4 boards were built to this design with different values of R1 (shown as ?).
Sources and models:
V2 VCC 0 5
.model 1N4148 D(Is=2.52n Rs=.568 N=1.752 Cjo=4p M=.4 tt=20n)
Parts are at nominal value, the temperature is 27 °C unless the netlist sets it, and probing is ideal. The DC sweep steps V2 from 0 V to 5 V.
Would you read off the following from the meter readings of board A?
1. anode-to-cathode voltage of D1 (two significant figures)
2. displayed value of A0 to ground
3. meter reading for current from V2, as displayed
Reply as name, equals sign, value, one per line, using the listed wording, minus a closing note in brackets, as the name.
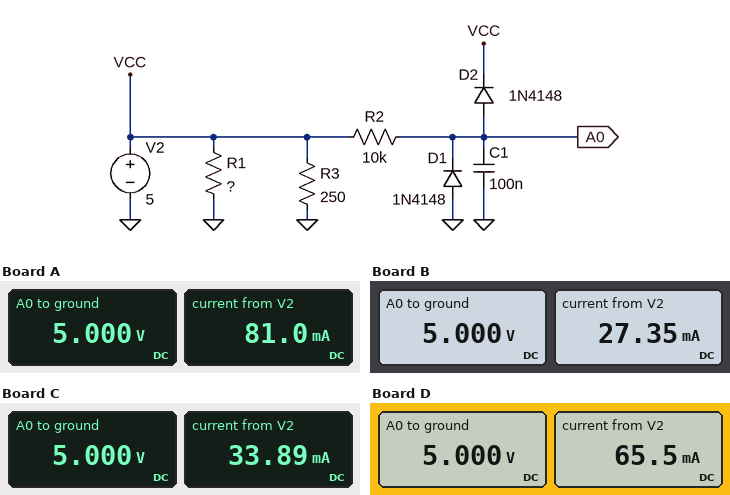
anode-to-cathode voltage of D1 = -5.0 V
displayed value of A0 to ground = 5.000 V
meter reading for current from V2, as displayed = 81.0 mA
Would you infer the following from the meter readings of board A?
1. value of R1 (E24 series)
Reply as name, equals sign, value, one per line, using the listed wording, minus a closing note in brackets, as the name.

value of R1 = 82 Ω
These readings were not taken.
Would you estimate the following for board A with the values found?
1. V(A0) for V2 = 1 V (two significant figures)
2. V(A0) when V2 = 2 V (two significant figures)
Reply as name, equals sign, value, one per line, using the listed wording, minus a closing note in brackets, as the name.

V(A0) for V2 = 1 V = 1.0 V
V(A0) when V2 = 2 V = 2.0 V
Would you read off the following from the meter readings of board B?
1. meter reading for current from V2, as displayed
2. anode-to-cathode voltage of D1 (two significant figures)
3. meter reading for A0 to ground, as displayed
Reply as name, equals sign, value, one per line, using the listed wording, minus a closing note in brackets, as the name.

meter reading for current from V2, as displayed = 27.35 mA
anode-to-cathode voltage of D1 = -5.0 V
meter reading for A0 to ground, as displayed = 5.000 V
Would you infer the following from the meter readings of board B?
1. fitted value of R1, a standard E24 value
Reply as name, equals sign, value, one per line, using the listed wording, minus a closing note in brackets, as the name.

fitted value of R1, a standard E24 value = 680 Ω
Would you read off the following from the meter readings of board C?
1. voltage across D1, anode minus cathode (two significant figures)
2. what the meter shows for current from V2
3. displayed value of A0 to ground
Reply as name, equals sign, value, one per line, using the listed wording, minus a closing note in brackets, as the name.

voltage across D1, anode minus cathode = -5.0 V
what the meter shows for current from V2 = 33.89 mA
displayed value of A0 to ground = 5.000 V
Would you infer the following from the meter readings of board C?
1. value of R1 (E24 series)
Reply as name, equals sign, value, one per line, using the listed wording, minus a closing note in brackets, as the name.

value of R1 = 360 Ω
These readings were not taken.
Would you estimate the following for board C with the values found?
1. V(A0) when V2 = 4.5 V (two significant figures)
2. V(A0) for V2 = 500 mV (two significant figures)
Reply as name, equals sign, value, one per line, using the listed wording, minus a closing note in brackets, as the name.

V(A0) when V2 = 4.5 V = 4.5 V
V(A0) for V2 = 500 mV = 500 mV
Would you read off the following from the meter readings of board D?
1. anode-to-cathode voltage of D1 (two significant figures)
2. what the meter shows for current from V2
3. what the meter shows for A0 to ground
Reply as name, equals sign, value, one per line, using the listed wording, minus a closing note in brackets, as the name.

anode-to-cathode voltage of D1 = -5.0 V
what the meter shows for current from V2 = 65.5 mA
what the meter shows for A0 to ground = 5.000 V
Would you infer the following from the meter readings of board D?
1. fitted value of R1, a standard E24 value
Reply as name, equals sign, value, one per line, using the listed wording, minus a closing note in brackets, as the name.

fitted value of R1, a standard E24 value = 110 Ω
